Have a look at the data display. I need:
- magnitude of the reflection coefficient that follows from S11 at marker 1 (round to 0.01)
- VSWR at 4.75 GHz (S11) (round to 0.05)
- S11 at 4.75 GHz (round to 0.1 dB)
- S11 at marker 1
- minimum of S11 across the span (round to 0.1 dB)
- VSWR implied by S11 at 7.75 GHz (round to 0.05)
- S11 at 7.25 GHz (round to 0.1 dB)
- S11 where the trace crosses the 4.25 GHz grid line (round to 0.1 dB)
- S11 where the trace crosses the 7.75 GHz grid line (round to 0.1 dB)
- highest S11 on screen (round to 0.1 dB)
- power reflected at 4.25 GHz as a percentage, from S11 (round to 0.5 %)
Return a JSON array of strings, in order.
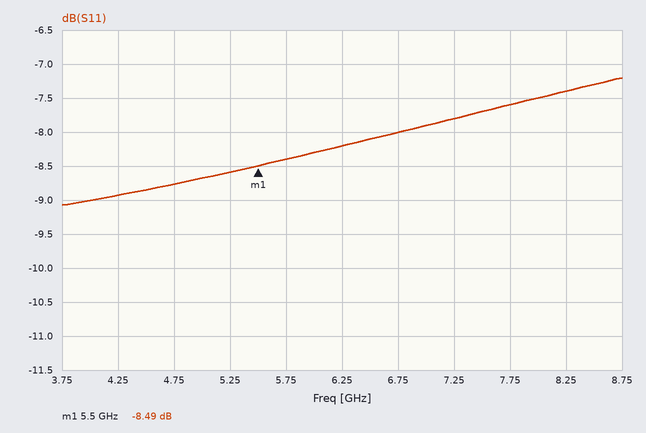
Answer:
["0.38", "2.15", "-8.8 dB", "-8.49 dB", "-9.1 dB", "2.45", "-7.8 dB", "-8.9 dB", "-7.6 dB", "-7.2 dB", "13.0 %"]
